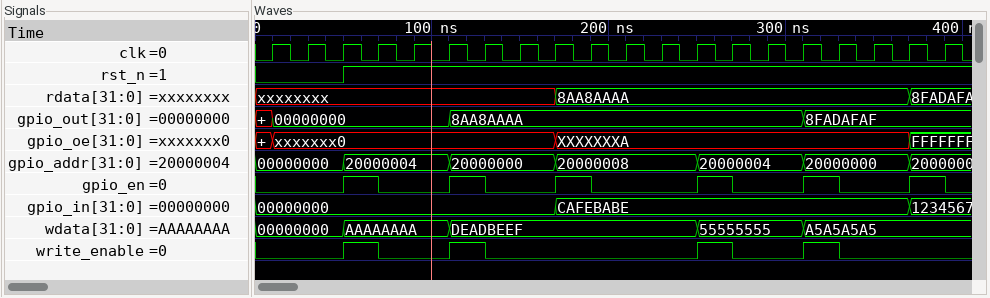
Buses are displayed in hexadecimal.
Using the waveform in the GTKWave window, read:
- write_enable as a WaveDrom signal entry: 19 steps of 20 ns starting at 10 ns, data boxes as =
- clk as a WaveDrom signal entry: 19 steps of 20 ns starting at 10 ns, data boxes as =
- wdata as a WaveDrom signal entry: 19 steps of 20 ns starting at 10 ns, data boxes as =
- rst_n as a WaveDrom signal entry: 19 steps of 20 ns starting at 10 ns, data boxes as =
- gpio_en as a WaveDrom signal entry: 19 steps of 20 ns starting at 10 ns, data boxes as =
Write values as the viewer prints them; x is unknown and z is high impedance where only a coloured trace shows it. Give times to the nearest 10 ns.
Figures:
{name: 'write_enable', wave: '0.10.10.....10.10..'}
{name: 'clk', wave: 'p..................'}
{name: 'wdata', wave: '=.=..=......=..=...', data: '00000000 AAAAAAAA DEADBEEF 55555555 A5A5A5A5'}
{name: 'rst_n', wave: '0.1................'}
{name: 'gpio_en', wave: '0.10.10.10..10.10.1'}
